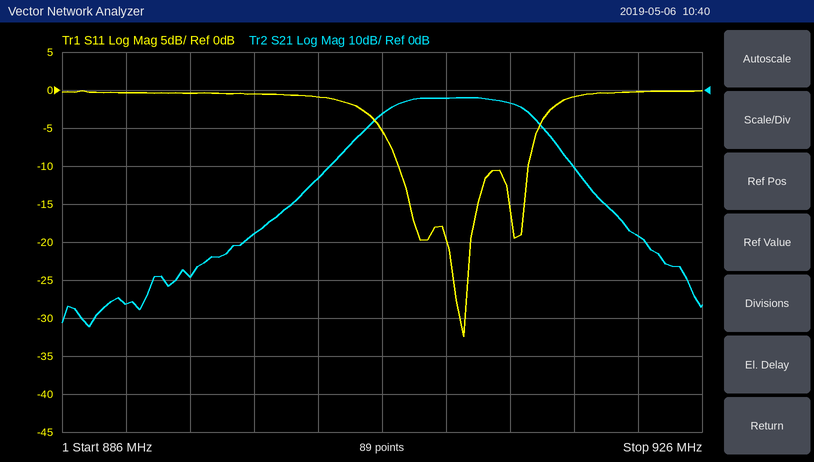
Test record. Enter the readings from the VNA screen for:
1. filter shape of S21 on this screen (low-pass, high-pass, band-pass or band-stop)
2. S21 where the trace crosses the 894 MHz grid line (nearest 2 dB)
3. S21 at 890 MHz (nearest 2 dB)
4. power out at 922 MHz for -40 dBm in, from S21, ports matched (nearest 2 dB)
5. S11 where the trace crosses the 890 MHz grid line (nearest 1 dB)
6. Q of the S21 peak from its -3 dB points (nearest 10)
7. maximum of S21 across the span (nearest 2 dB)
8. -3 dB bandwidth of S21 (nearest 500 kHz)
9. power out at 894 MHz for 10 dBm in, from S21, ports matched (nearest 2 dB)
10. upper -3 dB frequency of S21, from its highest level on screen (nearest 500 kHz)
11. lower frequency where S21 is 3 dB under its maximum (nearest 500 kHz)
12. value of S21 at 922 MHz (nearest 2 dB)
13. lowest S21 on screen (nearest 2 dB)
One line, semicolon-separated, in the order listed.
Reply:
band-pass; -50 dB; -56 dB; -78 dBm; 0 dB; 110; -2 dB; 8.5 MHz; -40 dBm; 915.0 MHz; 906.5 MHz; -38 dB; -62 dB
